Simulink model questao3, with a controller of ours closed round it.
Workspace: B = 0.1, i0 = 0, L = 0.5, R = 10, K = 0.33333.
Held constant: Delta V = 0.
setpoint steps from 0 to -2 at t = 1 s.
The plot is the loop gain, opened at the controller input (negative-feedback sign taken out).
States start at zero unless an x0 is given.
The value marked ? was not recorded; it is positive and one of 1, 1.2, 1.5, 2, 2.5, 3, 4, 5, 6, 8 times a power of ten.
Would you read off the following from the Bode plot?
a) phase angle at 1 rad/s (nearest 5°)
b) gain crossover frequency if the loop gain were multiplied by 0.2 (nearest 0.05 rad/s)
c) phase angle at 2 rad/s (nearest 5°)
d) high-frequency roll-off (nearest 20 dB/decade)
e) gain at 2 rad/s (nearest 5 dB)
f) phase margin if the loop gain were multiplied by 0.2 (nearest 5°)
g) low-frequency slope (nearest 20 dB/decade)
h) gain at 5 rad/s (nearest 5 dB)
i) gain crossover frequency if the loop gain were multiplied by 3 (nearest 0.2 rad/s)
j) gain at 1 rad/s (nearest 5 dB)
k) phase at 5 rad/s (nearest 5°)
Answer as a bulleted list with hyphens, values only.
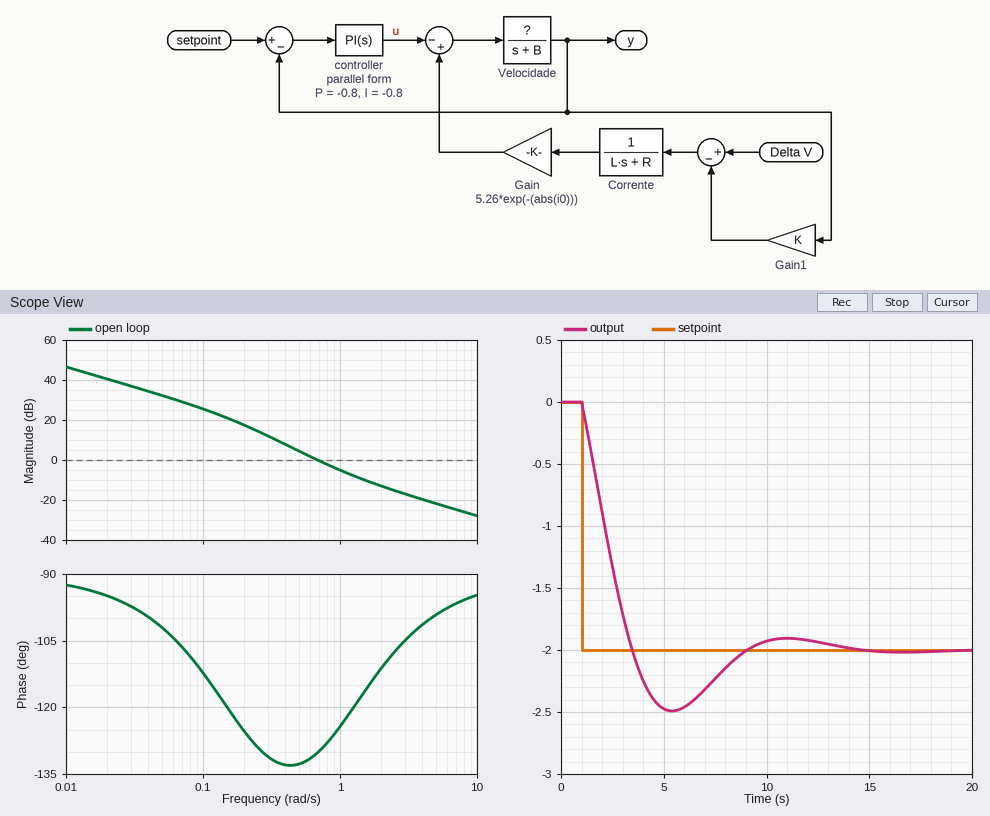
- -125°
- 0.25 rad/s
- -110°
- -20 dB/decade
- -15 dB
- 50°
- -20 dB/decade
- -20 dB
- 1.4 rad/s
- -5 dB
- -100°
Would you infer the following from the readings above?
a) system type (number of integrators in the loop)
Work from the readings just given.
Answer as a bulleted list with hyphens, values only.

- 1
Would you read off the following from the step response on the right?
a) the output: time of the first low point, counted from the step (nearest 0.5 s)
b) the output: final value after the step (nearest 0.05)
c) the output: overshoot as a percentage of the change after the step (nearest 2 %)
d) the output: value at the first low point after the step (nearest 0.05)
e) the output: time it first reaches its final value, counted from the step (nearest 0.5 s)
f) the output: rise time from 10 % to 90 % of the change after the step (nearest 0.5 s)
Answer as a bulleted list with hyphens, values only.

- 4.5 s
- -2.00
- 24 %
- -2.50
- 2.5 s
- 2.0 s
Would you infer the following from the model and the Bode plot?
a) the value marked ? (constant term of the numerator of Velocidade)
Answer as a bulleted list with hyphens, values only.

- 0.5
